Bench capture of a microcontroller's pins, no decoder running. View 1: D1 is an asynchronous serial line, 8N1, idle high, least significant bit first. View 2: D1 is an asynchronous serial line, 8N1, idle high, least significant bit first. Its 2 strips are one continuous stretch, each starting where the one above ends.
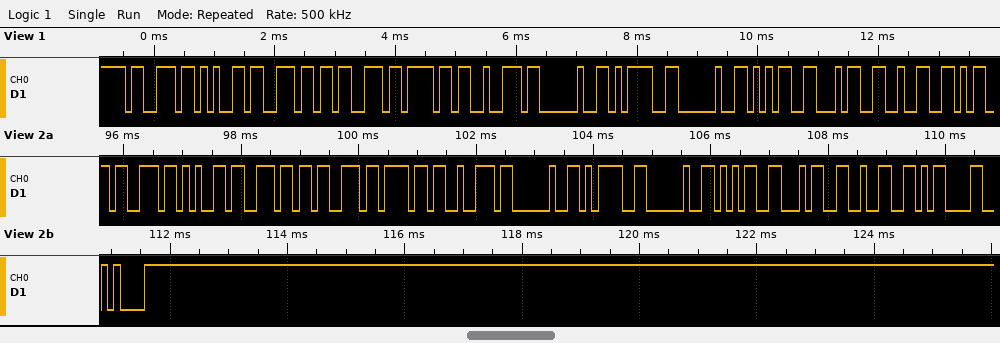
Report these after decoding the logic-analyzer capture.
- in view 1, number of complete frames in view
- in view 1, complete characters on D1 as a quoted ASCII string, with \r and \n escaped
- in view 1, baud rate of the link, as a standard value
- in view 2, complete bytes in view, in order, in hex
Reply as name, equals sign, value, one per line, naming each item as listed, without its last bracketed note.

in view 1, number of complete frames in view = 12
in view 1, complete characters on D1 as a quoted ASCII string, with \r and \n escaped = "sensor = 542"
in view 1, baud rate of the link, as a standard value = 9600 baud
in view 2, complete bytes in view, in order, in hex = 73 65 6E 73 6F 72 20 3D 20 35 34 32 0D 0A
